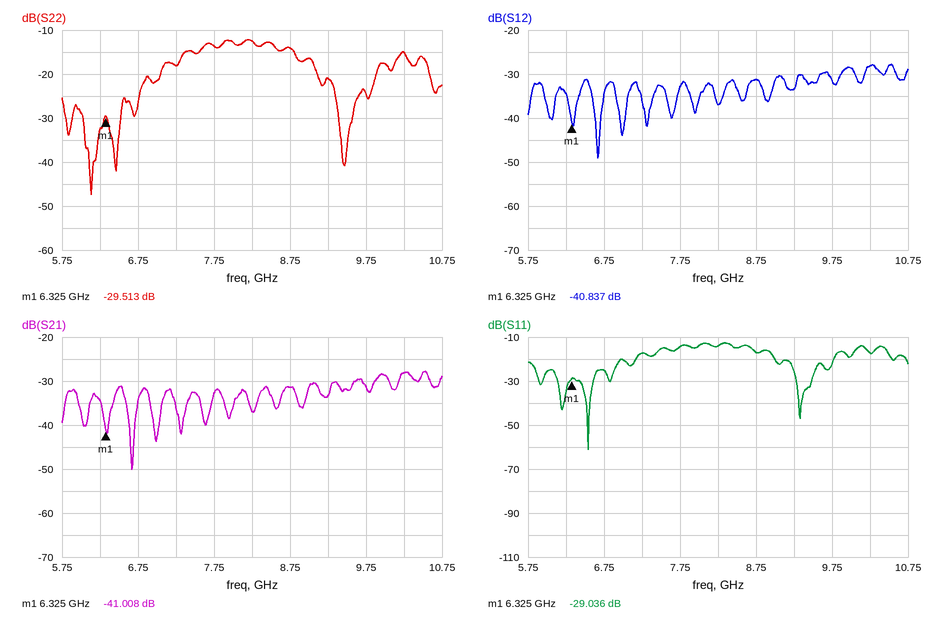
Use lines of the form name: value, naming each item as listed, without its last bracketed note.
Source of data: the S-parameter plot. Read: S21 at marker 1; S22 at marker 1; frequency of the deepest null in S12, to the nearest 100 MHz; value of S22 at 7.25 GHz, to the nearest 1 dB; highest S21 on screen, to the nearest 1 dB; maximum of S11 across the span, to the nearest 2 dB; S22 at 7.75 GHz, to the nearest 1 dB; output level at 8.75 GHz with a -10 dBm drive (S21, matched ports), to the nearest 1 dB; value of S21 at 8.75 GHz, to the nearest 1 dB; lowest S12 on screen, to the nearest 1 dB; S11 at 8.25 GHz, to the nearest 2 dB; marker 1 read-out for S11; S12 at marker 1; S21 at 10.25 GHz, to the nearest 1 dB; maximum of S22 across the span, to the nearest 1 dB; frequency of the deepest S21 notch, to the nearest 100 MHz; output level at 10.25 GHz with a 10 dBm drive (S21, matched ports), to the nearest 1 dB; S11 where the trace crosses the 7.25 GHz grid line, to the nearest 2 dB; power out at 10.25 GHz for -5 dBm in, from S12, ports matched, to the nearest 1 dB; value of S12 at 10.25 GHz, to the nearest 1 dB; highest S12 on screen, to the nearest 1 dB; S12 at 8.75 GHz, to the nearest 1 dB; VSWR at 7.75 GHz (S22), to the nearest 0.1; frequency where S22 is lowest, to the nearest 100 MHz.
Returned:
S21 at marker 1: -41.008 dB
S22 at marker 1: -29.513 dB
frequency of the deepest null in S12, to the nearest 100 MHz: 6.7 GHz
value of S22 at 7.25 GHz, to the nearest 1 dB: -18 dB
highest S21 on screen, to the nearest 1 dB: -28 dB
maximum of S11 across the span, to the nearest 2 dB: -12 dB
S22 at 7.75 GHz, to the nearest 1 dB: -14 dB
output level at 8.75 GHz with a -10 dBm drive (S21, matched ports), to the nearest 1 dB: -41 dBm
value of S21 at 8.75 GHz, to the nearest 1 dB: -31 dB
lowest S12 on screen, to the nearest 1 dB: -49 dB
S11 at 8.25 GHz, to the nearest 2 dB: -14 dB
marker 1 read-out for S11: -29.036 dB
S12 at marker 1: -40.837 dB
S21 at 10.25 GHz, to the nearest 1 dB: -28 dB
maximum of S22 across the span, to the nearest 1 dB: -12 dB
frequency of the deepest S21 notch, to the nearest 100 MHz: 6.7 GHz
output level at 10.25 GHz with a 10 dBm drive (S21, matched ports), to the nearest 1 dB: -18 dBm
S11 where the trace crosses the 7.25 GHz grid line, to the nearest 2 dB: -18 dB
power out at 10.25 GHz for -5 dBm in, from S12, ports matched, to the nearest 1 dB: -33 dBm
value of S12 at 10.25 GHz, to the nearest 1 dB: -28 dB
highest S12 on screen, to the nearest 1 dB: -28 dB
S12 at 8.75 GHz, to the nearest 1 dB: -31 dB
VSWR at 7.75 GHz (S22), to the nearest 0.1: 1.5
frequency where S22 is lowest, to the nearest 100 MHz: 6.1 GHz
